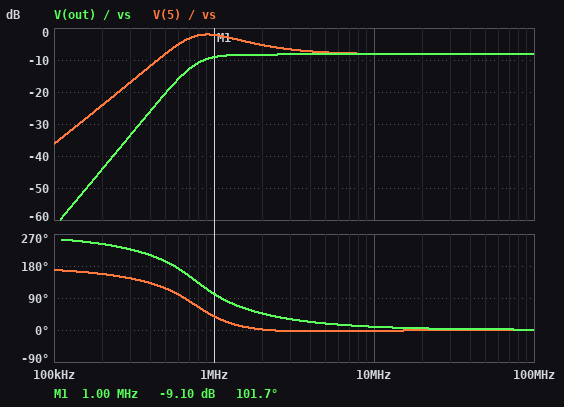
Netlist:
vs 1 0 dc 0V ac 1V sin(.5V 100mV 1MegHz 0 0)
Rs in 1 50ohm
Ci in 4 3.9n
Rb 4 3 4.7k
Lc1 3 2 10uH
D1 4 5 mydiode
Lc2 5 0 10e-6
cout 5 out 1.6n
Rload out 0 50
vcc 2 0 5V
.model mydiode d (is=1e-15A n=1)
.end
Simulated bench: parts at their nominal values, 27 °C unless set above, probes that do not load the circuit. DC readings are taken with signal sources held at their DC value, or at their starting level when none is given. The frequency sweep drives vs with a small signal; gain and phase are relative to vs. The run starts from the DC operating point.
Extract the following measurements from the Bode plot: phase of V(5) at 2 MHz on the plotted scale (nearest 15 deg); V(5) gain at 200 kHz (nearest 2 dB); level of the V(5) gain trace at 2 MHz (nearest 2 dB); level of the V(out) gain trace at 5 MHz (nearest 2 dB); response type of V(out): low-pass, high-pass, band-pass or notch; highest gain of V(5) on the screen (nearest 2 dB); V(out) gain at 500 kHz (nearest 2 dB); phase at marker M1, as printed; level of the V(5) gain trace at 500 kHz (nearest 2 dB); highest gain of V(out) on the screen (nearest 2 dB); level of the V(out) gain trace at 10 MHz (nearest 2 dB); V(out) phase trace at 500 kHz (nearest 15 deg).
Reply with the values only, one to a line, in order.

0 deg
-24 dB
-6 dB
-8 dB
high-pass
-2 dB
-20 dB
101.7 deg
-8 dB
-8 dB
-8 dB
195 deg
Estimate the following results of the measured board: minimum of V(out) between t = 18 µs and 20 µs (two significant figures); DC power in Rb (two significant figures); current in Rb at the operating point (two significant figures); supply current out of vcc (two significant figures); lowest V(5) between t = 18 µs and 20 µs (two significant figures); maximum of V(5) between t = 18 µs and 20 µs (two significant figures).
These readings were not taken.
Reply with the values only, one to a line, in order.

-35 mV
3.9 mW
910 µA
910 µA
-78 mV
75 mV
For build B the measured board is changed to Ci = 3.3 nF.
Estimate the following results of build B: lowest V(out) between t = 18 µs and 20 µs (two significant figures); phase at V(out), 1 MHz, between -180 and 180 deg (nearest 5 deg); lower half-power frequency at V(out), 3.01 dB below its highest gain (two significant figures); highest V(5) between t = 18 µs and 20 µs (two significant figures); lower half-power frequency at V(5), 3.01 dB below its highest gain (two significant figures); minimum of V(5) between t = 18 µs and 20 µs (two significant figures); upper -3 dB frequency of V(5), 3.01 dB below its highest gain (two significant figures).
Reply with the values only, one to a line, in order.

-36 mV
105 deg
770 kHz
76 mV
630 kHz
-79 mV
1.8 MHz
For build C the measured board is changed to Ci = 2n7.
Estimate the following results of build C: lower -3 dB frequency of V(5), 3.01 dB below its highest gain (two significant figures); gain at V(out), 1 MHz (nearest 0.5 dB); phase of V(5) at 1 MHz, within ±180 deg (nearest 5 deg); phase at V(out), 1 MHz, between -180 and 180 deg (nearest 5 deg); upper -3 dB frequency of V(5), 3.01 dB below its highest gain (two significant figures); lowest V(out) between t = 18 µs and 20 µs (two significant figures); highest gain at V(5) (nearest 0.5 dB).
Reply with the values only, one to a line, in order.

660 kHz
-8.5 dB
45 deg
110 deg
1.7 MHz
-37 mV
-1.5 dB
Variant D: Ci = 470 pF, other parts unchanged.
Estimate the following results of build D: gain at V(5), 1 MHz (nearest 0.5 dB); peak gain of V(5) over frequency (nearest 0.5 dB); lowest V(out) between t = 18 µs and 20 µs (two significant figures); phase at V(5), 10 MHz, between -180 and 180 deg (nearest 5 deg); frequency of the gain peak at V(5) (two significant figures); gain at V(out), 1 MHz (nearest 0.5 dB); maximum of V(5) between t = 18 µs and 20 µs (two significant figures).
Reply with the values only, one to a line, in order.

-8.0 dB
-5.5 dB
-18 mV
10 deg
1.2 MHz
-15.0 dB
40 mV
